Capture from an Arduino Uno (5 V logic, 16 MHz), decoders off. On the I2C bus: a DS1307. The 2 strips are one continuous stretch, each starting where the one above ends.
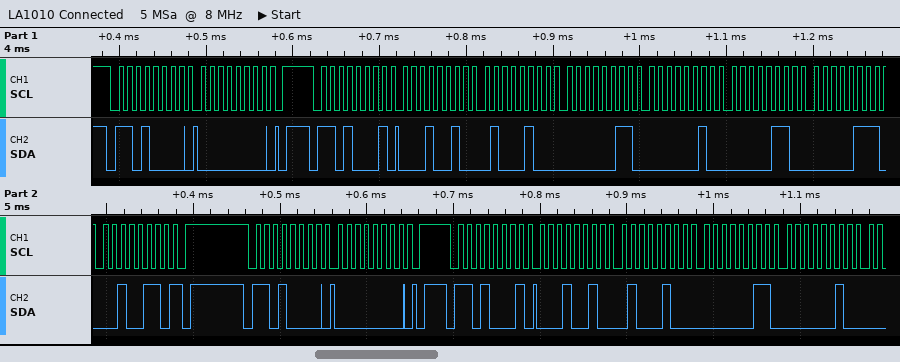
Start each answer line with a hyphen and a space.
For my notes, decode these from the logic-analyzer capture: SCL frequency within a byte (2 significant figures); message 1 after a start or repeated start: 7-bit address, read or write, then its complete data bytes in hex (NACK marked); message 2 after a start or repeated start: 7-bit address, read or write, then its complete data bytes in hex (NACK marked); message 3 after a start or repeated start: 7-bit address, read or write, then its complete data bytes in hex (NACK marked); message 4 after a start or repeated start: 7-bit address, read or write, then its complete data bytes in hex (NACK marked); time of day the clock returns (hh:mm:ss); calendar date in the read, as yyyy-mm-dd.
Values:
- 100 kHz
- 0x68 write: 00
- 0x68 read: 12 44 03 02 06 07 26 NACK
- 0x68 write: 00
- 0x68 read: 12 44 03 02
- 03:44:12
- 2026-07-06
